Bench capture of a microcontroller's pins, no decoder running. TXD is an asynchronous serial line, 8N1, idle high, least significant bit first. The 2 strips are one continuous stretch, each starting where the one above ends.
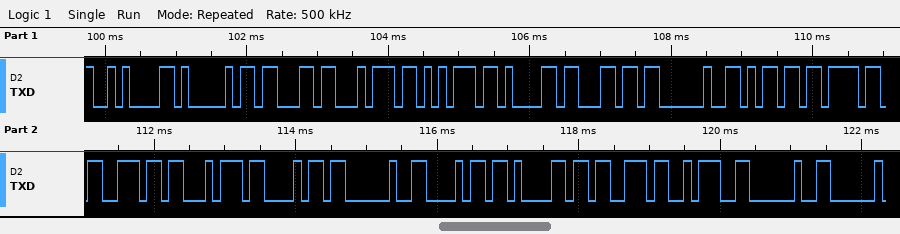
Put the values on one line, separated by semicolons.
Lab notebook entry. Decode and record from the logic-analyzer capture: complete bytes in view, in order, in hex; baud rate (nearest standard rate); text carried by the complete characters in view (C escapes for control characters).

0A 41 63 74 75 61 6C 20 6D 6F 6E 74 68 20 68 61 73 3A 20; 9600 baud; "\nActual month has: "
